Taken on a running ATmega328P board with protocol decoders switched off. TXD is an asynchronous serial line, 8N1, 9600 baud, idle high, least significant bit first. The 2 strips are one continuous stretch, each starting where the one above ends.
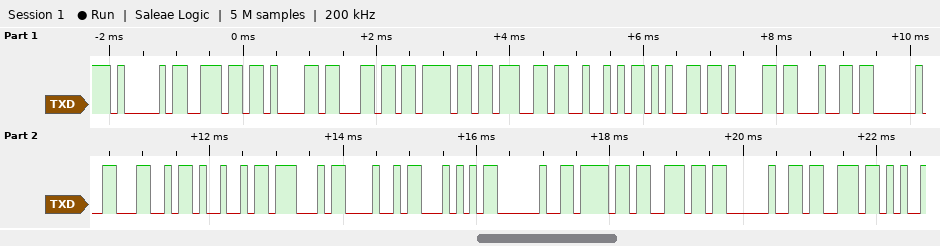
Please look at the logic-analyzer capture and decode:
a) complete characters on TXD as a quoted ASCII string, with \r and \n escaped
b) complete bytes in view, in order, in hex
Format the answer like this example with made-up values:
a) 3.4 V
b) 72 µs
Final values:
a) "AnalogRead LIGHT on s"
b) 41 6E 61 6C 6F 67 52 65 61 64 20 4C 49 47 48 54 20 6F 6E 20 73
